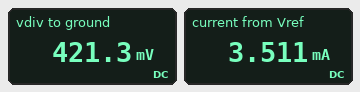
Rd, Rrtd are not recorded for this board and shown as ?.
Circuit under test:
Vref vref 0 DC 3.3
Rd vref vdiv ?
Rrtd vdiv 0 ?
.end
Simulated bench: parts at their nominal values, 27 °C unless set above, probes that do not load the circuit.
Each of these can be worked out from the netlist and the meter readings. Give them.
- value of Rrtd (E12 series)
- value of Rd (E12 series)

120 Ω
820 Ω
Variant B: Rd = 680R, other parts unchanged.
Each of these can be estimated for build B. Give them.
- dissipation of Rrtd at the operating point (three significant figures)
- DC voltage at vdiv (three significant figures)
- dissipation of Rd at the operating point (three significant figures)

2.04 mW
495 mV
11.6 mW
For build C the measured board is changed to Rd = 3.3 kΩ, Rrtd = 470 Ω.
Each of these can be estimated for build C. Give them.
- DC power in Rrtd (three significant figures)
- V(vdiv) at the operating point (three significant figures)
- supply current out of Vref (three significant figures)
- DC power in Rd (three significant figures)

360 µW
411 mV
875 µA
2.53 mW
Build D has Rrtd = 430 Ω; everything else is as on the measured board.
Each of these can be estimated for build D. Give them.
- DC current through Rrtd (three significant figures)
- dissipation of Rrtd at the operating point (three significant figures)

2.64 mA
3.00 mW
